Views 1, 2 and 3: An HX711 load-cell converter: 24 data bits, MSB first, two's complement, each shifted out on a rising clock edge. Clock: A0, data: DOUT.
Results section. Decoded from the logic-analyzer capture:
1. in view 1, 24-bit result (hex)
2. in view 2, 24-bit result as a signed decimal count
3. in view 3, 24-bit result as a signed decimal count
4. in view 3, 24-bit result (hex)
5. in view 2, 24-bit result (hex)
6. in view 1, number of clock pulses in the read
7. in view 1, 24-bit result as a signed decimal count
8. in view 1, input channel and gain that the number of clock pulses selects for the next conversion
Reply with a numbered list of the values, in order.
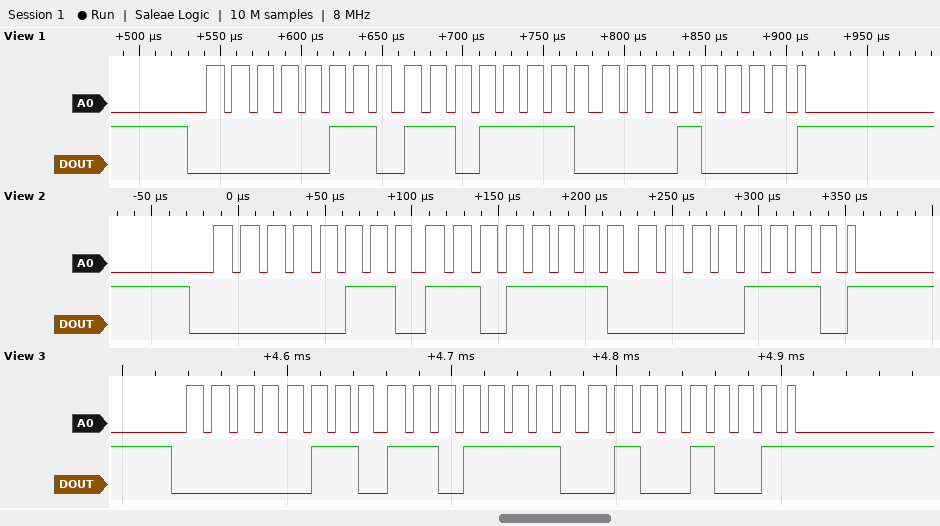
1. 0x06DE10
2. 450062
3. 450121
4. 0x06DE49
5. 0x06DE0E
6. 25
7. 450064
8. channel A, gain 128
